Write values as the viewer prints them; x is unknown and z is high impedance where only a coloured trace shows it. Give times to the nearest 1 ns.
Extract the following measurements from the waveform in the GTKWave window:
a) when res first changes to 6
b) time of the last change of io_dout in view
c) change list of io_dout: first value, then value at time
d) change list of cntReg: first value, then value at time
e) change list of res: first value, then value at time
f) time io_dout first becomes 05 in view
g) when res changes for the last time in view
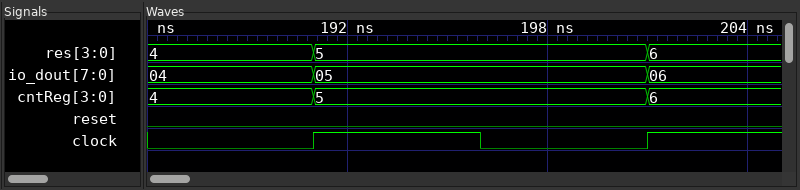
201 ns
201 ns
04, 05 at 191 ns, 06 at 201 ns
4, 5 at 191 ns, 6 at 201 ns
4, 5 at 191 ns, 6 at 201 ns
191 ns
201 ns
